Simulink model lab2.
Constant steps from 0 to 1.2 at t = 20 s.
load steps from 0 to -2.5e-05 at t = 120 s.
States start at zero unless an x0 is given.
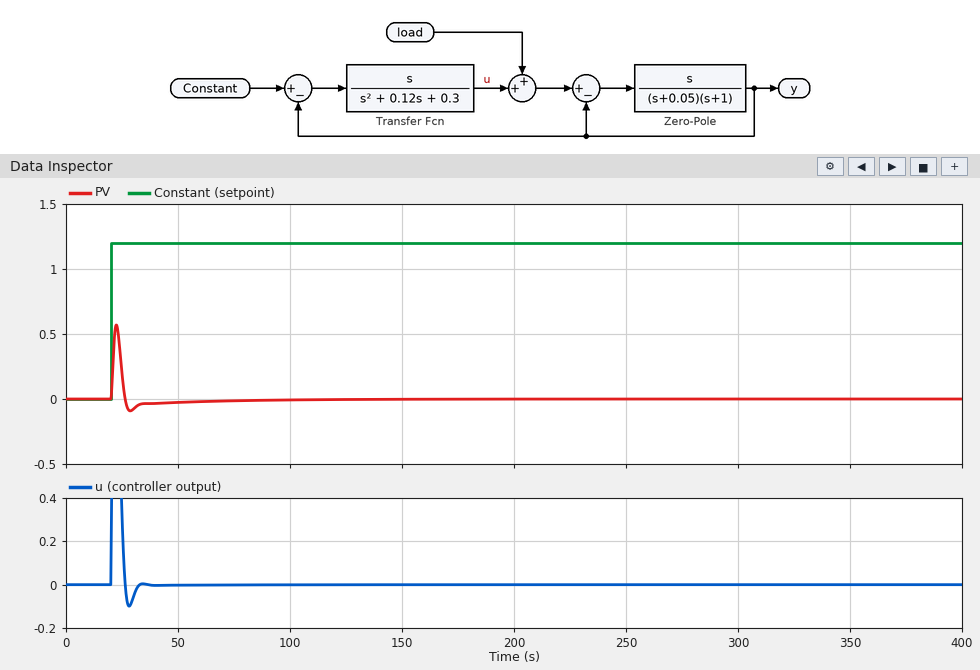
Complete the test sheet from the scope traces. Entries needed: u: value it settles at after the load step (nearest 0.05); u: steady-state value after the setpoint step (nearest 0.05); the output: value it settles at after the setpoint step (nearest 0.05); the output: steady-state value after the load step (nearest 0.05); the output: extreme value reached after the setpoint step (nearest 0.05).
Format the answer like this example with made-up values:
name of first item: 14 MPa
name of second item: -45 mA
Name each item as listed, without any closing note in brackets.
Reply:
u: value it settles at after the load step: 0.00
u: steady-state value after the setpoint step: 0.00
the output: value it settles at after the setpoint step: 0.00
the output: steady-state value after the load step: 0.00
the output: extreme value reached after the setpoint step: 0.55
